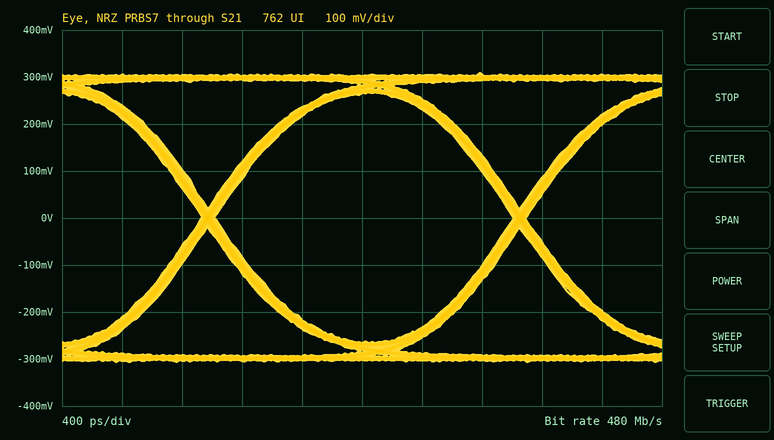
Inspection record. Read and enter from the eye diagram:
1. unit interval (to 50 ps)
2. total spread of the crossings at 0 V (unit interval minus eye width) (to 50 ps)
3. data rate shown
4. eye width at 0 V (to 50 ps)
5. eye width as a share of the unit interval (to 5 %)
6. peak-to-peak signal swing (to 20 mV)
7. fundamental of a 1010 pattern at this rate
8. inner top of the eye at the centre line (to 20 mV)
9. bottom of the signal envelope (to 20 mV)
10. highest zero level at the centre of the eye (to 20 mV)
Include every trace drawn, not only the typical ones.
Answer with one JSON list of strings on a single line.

["2.10 ns", "100 ps", "480 Mb/s", "2.00 ns", "95 %", "620 mV", "240 MHz", "260 mV", "-300 mV", "-260 mV"]
